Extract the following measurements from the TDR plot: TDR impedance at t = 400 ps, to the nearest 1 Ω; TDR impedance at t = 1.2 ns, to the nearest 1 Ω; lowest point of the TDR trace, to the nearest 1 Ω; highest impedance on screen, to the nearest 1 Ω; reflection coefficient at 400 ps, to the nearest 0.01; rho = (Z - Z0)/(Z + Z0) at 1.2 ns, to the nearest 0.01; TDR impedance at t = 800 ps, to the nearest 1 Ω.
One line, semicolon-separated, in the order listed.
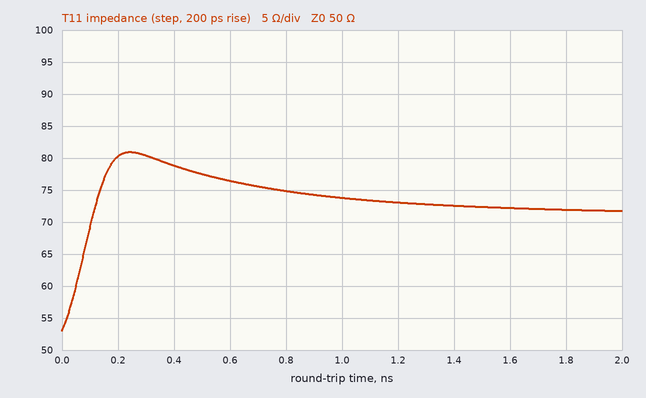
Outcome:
79 Ω; 73 Ω; 53 Ω; 81 Ω; +0.22; +0.19; 75 Ω
